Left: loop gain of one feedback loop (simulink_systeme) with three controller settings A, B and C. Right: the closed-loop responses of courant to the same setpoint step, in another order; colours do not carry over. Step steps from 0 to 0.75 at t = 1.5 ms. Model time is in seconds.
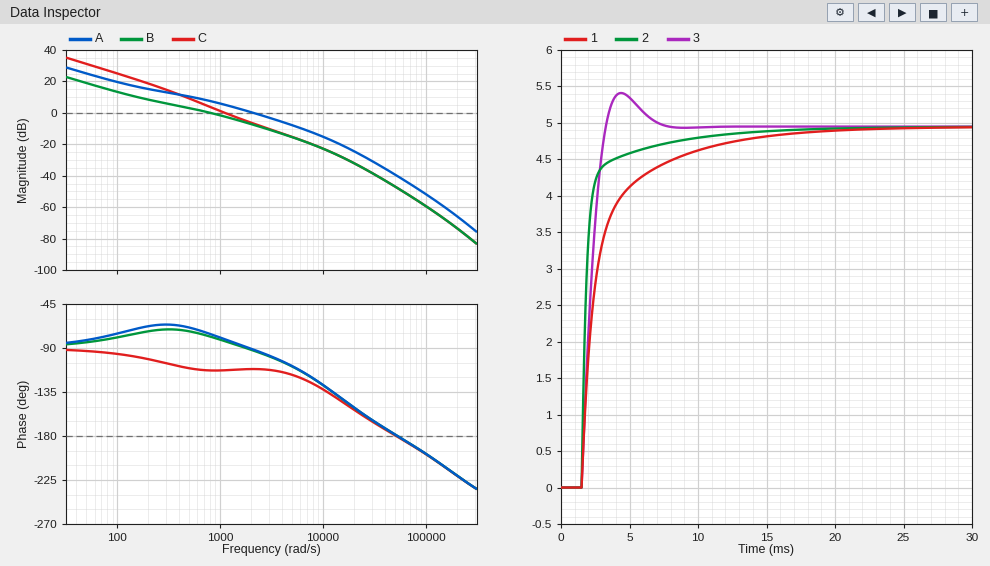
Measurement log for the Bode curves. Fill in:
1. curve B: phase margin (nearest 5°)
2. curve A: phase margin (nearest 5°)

100°
90°
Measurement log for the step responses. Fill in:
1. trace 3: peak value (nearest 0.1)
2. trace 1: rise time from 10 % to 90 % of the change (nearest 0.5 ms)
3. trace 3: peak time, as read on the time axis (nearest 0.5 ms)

5.4
6.0 ms
4.5 ms
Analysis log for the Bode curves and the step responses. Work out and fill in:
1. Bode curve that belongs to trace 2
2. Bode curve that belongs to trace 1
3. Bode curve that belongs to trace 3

A
B
C
